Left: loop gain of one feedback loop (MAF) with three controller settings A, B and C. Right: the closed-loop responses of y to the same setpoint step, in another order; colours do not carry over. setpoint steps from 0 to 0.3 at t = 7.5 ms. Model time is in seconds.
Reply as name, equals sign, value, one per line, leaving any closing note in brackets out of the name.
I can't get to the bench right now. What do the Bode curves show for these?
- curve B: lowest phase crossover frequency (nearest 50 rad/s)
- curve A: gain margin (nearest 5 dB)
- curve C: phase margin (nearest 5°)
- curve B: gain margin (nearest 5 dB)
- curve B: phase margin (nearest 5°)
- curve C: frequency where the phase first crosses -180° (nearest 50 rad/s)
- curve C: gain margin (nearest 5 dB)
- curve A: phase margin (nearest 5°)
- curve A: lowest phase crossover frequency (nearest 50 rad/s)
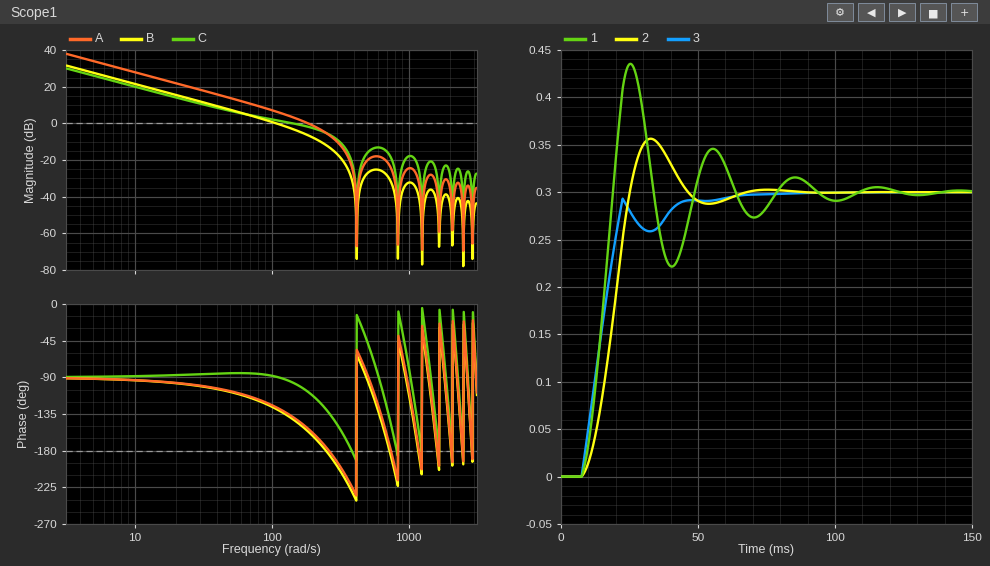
curve B: lowest phase crossover frequency = 250 rad/s
curve A: gain margin = 5 dB
curve C: phase margin = 85°
curve B: gain margin = 10 dB
curve B: phase margin = 50°
curve C: frequency where the phase first crosses -180° = 400 rad/s
curve C: gain margin = 20 dB
curve A: phase margin = 25°
curve A: lowest phase crossover frequency = 250 rad/s
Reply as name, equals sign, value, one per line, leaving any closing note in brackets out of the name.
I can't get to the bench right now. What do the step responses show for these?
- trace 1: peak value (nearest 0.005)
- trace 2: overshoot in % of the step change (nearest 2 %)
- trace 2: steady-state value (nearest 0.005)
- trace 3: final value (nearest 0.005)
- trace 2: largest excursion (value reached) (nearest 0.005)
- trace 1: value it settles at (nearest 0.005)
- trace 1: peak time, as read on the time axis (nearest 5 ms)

trace 1: peak value = 0.435
trace 2: overshoot in % of the step change = 18 %
trace 2: steady-state value = 0.300
trace 3: final value = 0.300
trace 2: largest excursion (value reached) = 0.355
trace 1: value it settles at = 0.300
trace 1: peak time, as read on the time axis = 25 ms
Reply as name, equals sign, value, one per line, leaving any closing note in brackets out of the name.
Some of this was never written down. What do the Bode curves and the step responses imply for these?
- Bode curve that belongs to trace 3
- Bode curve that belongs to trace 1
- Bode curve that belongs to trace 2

Bode curve that belongs to trace 3 = C
Bode curve that belongs to trace 1 = A
Bode curve that belongs to trace 2 = B
